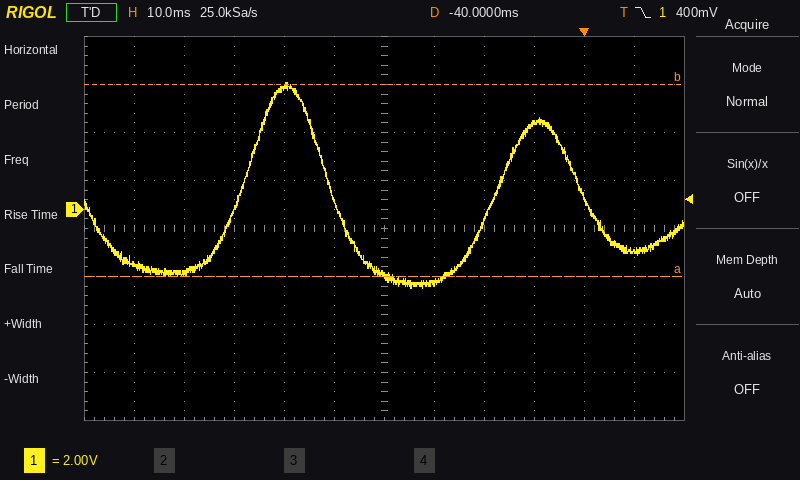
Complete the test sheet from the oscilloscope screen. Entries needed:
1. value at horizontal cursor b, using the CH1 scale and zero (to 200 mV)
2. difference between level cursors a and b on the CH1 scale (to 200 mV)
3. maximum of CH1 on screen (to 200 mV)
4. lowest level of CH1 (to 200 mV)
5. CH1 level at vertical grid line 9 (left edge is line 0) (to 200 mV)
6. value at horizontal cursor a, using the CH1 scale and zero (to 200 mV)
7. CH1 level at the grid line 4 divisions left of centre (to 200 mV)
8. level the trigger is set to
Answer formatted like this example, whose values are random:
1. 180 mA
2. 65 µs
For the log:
1. 5.2 V
2. 8.0 V
3. 5.2 V
4. -3.2 V
5. 3.6 V
6. -2.8 V
7. -2.6 V
8. 400 mV
